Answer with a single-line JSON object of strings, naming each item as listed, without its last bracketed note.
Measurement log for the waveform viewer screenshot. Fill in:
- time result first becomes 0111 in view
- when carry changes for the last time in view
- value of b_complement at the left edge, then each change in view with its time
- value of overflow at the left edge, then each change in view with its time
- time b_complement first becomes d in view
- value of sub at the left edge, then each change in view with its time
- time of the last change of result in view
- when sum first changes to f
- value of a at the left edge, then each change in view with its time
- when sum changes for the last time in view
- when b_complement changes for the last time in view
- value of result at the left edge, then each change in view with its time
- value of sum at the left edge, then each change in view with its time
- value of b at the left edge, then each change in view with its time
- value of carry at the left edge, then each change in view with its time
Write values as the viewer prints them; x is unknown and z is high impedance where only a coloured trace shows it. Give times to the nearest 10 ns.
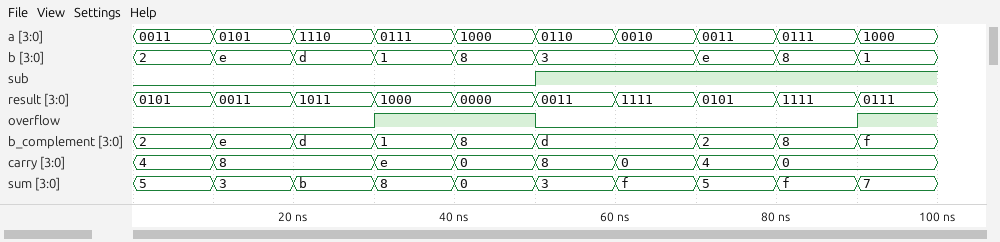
{"time result first becomes 0111 in view": "90 ns", "when carry changes for the last time in view": "80 ns", "value of b_complement at the left edge, then each change in view with its time": "2, e at 10 ns, d at 20 ns, 1 at 30 ns, 8 at 40 ns, d at 50 ns, 2 at 70 ns, 8 at 80 ns, f at 90 ns", "value of overflow at the left edge, then each change in view with its time": "0, 1 at 30 ns, 0 at 50 ns, 1 at 90 ns", "time b_complement first becomes d in view": "20 ns", "value of sub at the left edge, then each change in view with its time": "0, 1 at 50 ns", "time of the last change of result in view": "90 ns", "when sum first changes to f": "60 ns", "value of a at the left edge, then each change in view with its time": "0011, 0101 at 10 ns, 1110 at 20 ns, 0111 at 30 ns, 1000 at 40 ns, 0110 at 50 ns, 0010 at 60 ns, 0011 at 70 ns, 0111 at 80 ns, 1000 at 90 ns", "when sum changes for the last time in view": "90 ns", "when b_complement changes for the last time in view": "90 ns", "value of result at the left edge, then each change in view with its time": "0101, 0011 at 10 ns, 1011 at 20 ns, 1000 at 30 ns, 0000 at 40 ns, 0011 at 50 ns, 1111 at 60 ns, 0101 at 70 ns, 1111 at 80 ns, 0111 at 90 ns", "value of sum at the left edge, then each change in view with its time": "5, 3 at 10 ns, b at 20 ns, 8 at 30 ns, 0 at 40 ns, 3 at 50 ns, f at 60 ns, 5 at 70 ns, f at 80 ns, 7 at 90 ns", "value of b at the left edge, then each change in view with its time": "2, e at 10 ns, d at 20 ns, 1 at 30 ns, 8 at 40 ns, 3 at 50 ns, e at 70 ns, 8 at 80 ns, 1 at 90 ns", "value of carry at the left edge, then each change in view with its time": "4, 8 at 10 ns, e at 30 ns, 0 at 40 ns, 8 at 50 ns, 0 at 60 ns, 4 at 70 ns, 0 at 80 ns"}
